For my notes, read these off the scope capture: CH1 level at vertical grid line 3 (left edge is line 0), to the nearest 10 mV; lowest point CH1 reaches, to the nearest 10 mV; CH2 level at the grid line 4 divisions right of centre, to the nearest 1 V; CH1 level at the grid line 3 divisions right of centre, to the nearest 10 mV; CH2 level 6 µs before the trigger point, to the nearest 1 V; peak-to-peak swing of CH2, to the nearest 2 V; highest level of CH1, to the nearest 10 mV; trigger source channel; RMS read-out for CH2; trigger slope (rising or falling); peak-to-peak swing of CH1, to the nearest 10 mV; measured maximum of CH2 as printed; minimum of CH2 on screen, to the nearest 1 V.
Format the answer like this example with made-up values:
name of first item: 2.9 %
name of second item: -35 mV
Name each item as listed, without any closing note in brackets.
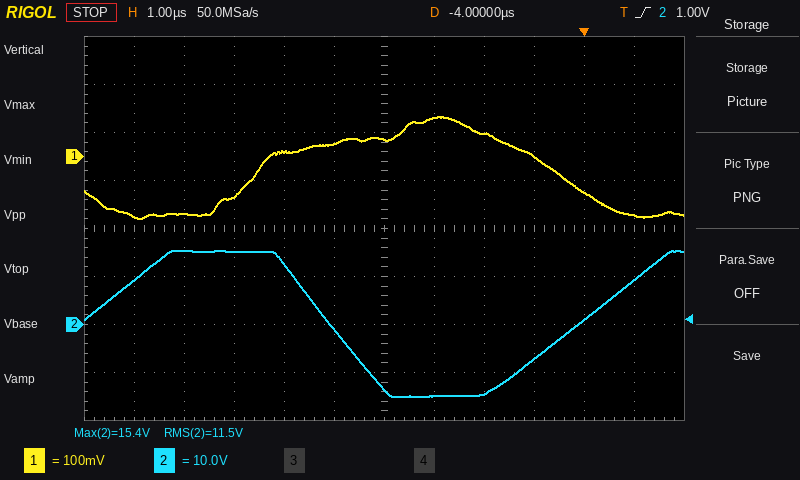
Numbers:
CH1 level at vertical grid line 3 (left edge is line 0), to the nearest 10 mV: -80 mV
lowest point CH1 reaches, to the nearest 10 mV: -130 mV
CH2 level at the grid line 4 divisions right of centre, to the nearest 1 V: 1 V
CH1 level at the grid line 3 divisions right of centre, to the nearest 10 mV: 0 mV
CH2 level 6 µs before the trigger point, to the nearest 1 V: 13 V
peak-to-peak swing of CH2, to the nearest 2 V: 30 V
highest level of CH1, to the nearest 10 mV: 80 mV
trigger source channel: CH2
RMS read-out for CH2: 11.5 V
trigger slope: rising
peak-to-peak swing of CH1, to the nearest 10 mV: 210 mV
measured maximum of CH2 as printed: 15.4 V
minimum of CH2 on screen, to the nearest 1 V: -15 V
